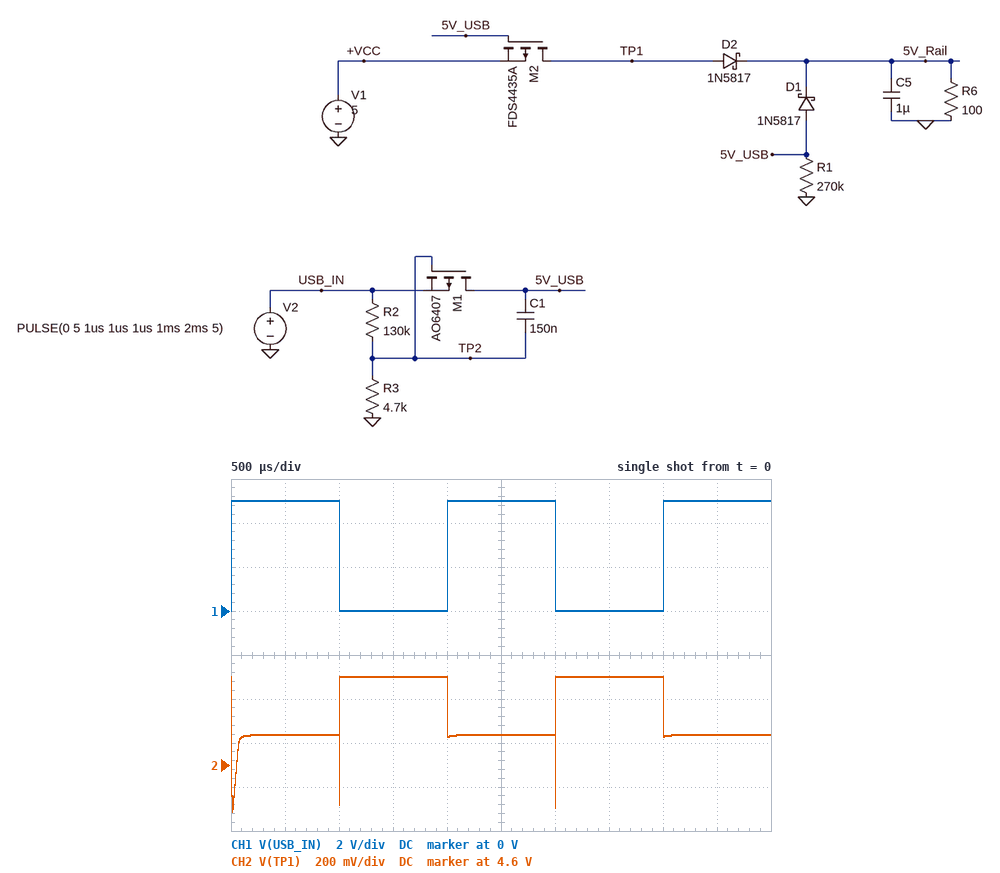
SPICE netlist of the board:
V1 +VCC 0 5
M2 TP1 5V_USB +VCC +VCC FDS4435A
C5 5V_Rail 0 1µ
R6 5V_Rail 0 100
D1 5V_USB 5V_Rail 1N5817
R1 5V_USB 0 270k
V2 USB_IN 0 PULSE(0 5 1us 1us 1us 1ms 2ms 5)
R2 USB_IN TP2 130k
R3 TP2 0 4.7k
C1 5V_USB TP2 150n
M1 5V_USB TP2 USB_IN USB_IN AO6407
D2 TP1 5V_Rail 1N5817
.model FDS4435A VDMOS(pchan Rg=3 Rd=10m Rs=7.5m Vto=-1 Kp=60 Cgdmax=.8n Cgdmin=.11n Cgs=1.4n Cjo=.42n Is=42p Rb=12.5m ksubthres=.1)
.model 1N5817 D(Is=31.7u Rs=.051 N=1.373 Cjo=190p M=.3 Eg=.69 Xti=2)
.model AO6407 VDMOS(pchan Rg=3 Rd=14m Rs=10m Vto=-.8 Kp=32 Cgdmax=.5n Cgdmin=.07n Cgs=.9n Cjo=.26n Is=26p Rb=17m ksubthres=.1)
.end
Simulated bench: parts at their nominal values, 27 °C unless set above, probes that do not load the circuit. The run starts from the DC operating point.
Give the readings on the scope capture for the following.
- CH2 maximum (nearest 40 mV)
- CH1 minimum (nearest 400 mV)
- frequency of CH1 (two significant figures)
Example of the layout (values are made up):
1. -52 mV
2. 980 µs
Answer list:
1. 5.00 V
2. 0 V
3. 500 Hz
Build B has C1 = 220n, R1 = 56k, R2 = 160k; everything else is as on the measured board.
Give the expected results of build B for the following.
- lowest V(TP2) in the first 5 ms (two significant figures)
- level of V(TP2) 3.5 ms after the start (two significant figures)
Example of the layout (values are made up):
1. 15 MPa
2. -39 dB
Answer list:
1. -3.5 V
2. -2.1 V
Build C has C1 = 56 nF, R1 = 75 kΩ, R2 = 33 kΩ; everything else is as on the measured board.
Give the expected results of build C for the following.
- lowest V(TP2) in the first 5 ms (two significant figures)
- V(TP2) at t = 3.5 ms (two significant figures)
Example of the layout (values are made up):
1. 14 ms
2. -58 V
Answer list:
1. -4.3 V
2. -520 mV
